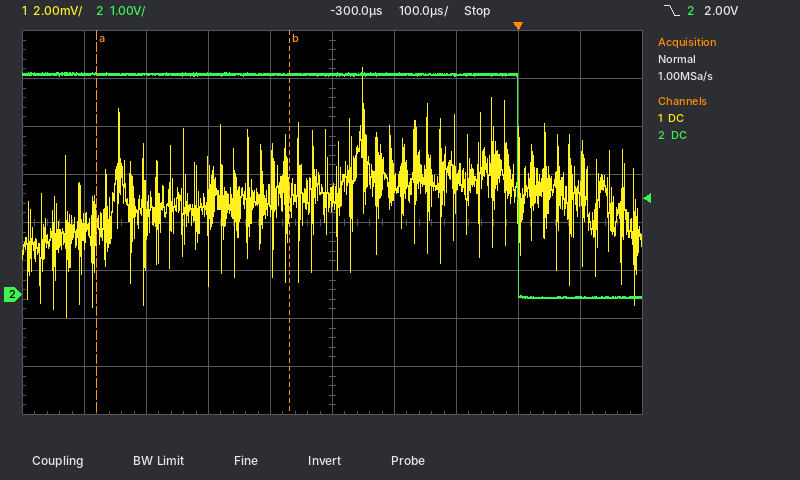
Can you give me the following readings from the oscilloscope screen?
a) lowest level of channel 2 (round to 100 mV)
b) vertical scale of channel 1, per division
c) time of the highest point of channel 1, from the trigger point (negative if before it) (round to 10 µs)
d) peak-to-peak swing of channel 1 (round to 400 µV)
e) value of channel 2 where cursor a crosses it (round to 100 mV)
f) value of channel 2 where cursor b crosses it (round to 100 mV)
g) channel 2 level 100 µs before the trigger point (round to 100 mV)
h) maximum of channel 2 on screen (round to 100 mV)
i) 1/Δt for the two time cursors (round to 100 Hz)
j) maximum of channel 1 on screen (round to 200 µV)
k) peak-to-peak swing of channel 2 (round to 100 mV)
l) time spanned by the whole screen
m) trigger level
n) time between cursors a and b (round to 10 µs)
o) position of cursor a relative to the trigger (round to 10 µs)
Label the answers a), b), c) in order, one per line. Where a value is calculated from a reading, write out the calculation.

a) -100 mV
b) 2 mV
c) -250 µs
d) 10.4 mV
e) 4.6 V
f) 4.6 V
g) 4.6 V
h) 4.6 V
i) 1 / 310 µs ≈ 3.2 kHz
j) 9.4 mV
k) 4.6 V − (-100 mV) = 4.7 V
l) 1 ms
m) 2.00 V
n) 310 µs
o) -680 µs
